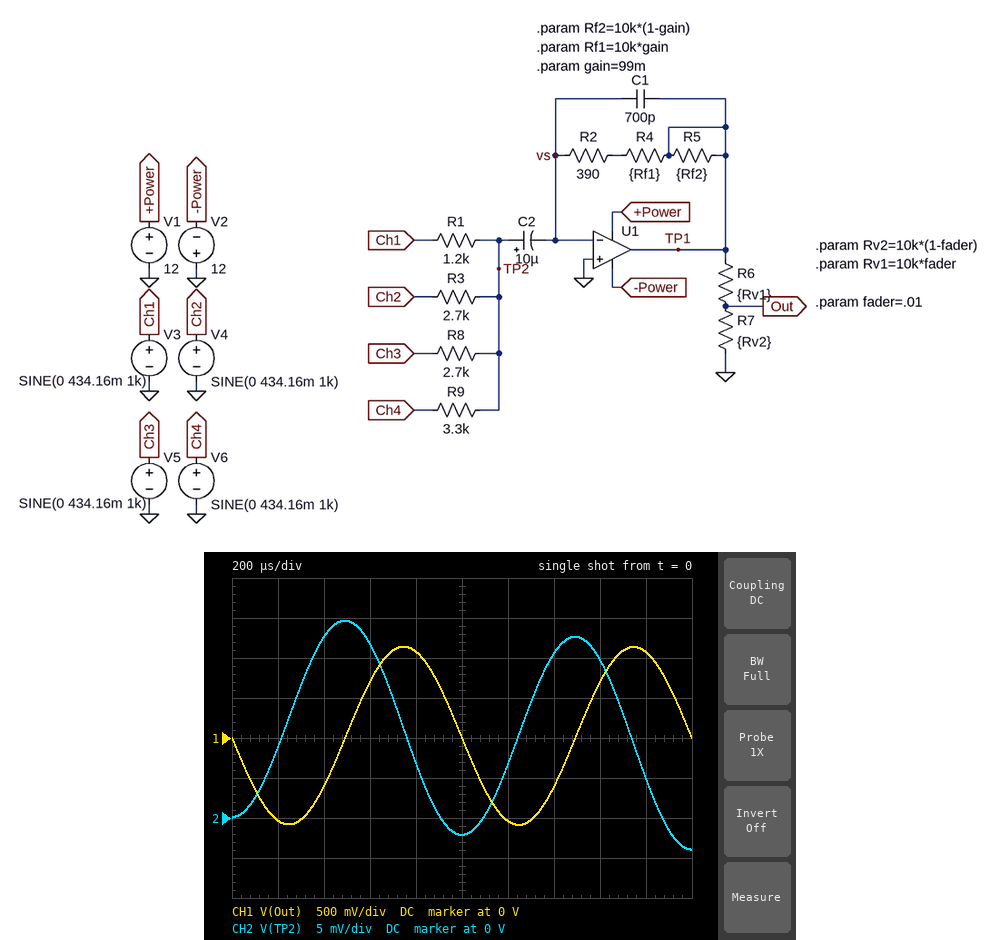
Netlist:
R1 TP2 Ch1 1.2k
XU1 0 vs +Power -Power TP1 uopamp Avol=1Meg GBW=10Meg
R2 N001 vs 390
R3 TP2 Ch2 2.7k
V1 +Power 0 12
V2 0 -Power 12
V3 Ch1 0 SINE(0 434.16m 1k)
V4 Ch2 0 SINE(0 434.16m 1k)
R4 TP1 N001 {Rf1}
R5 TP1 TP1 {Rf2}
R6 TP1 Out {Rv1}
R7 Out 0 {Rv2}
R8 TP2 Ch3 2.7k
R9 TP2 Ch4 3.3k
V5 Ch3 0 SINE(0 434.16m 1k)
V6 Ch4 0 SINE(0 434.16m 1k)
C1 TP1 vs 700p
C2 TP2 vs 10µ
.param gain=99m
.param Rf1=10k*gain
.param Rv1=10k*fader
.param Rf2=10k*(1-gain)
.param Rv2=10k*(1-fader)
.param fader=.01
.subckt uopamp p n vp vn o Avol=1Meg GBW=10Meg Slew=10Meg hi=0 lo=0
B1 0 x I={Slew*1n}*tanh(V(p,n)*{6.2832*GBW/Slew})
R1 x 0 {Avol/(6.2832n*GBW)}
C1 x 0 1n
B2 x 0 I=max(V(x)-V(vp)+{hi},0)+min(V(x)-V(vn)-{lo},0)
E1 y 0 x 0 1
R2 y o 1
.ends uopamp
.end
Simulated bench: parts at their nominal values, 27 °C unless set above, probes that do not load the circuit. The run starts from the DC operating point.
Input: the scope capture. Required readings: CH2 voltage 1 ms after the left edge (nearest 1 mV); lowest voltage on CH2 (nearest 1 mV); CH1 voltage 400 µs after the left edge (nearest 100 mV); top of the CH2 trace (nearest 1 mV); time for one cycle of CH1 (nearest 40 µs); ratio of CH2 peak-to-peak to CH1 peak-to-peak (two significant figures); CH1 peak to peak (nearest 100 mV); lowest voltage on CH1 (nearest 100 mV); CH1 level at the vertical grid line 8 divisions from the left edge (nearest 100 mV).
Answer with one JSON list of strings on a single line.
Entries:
["-2 mV", "-4 mV", "-600 mV", "25 mV", "1.00 ms", "0.013", "2.2 V", "-1.1 V", "700 mV"]
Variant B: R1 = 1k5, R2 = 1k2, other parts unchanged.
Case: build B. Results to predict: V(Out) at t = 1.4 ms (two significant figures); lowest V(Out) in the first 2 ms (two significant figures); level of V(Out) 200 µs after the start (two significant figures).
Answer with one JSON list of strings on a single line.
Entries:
["-890 mV", "-1.6 V", "-1.5 V"]
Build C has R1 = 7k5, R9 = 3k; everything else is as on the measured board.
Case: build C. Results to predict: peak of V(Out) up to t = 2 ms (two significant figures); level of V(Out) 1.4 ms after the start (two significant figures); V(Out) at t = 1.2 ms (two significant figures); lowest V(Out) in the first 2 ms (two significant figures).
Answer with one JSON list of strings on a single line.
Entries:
["730 mV", "-400 mV", "-670 mV", "-700 mV"]
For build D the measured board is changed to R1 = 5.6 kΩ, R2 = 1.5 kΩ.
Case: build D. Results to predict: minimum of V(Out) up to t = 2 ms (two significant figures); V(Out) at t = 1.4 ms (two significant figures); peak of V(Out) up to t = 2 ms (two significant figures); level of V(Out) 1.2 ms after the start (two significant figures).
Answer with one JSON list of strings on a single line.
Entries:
["-1.3 V", "-740 mV", "1.3 V", "-1.2 V"]
